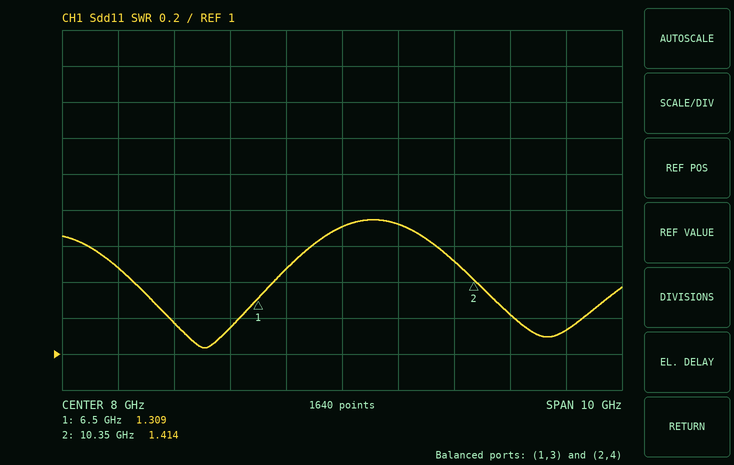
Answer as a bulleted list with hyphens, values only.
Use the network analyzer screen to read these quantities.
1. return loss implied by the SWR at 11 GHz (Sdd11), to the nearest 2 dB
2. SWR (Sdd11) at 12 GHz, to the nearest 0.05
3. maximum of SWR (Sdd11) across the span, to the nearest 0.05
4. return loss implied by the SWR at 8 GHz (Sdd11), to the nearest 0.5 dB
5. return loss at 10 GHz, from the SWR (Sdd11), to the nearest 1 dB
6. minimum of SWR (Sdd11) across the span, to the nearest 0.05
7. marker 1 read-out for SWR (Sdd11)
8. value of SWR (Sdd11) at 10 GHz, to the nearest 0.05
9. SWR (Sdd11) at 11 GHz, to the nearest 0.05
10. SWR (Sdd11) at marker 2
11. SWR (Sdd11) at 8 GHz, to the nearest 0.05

- 20 dB
- 1.15
- 1.75
- 11.5 dB
- 14 dB
- 1.05
- 1.309
- 1.50
- 1.20
- 1.414
- 1.70
